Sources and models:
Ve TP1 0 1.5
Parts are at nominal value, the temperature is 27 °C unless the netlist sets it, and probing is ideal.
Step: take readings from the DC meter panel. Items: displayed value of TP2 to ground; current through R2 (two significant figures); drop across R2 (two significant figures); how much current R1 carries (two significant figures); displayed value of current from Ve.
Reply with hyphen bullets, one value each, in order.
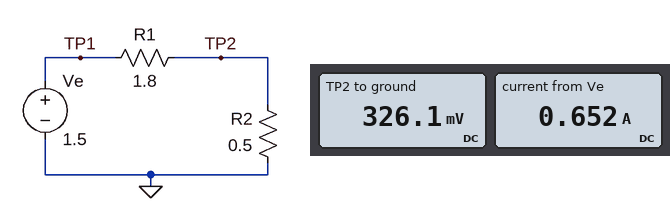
- 326.1 mV
- 650 mA
- 330 mV
- 650 mA
- 0.652 A
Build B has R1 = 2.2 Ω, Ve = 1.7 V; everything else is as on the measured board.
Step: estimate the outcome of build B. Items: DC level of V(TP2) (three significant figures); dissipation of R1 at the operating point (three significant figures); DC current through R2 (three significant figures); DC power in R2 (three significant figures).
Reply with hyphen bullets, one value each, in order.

- 315 mV
- 872 mW
- 630 mA
- 198 mW
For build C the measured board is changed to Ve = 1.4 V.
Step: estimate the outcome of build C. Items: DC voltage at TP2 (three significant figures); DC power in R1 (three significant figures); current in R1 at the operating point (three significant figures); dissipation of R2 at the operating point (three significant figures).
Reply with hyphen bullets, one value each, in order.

- 304 mV
- 667 mW
- 609 mA
- 185 mW
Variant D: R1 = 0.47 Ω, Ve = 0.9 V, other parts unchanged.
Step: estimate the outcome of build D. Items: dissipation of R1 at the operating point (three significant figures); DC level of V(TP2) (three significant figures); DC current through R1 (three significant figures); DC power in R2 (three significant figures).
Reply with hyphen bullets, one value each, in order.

- 405 mW
- 464 mV
- 928 mA
- 430 mW
